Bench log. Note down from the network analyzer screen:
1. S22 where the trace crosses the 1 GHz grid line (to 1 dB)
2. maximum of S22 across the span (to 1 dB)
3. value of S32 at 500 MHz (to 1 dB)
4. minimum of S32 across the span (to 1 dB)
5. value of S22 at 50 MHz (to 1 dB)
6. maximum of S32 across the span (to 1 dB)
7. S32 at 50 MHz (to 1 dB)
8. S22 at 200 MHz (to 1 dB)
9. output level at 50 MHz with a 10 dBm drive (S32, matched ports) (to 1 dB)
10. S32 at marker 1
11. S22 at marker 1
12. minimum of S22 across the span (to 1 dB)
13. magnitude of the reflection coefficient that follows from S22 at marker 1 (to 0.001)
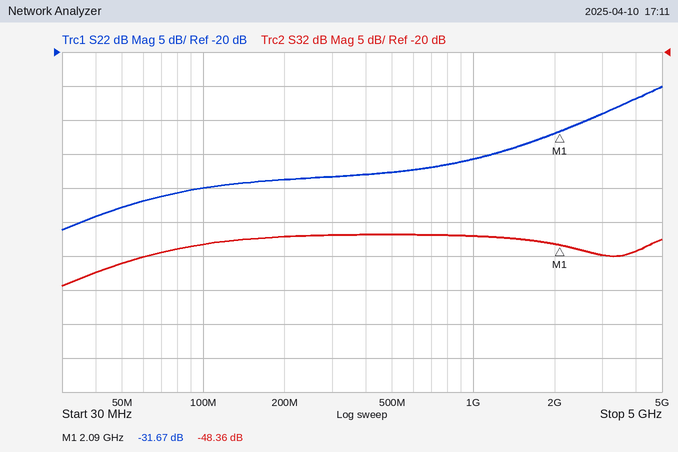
-36 dB
-25 dB
-47 dB
-54 dB
-43 dB
-47 dB
-51 dB
-39 dB
-41 dBm
-48.36 dB
-31.67 dB
-46 dB
0.026
